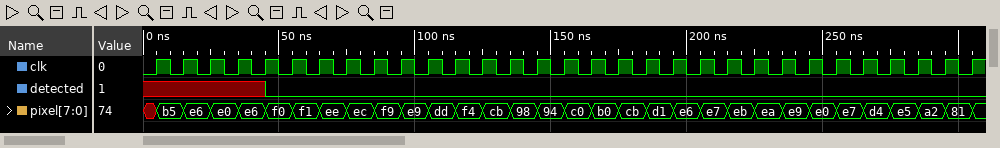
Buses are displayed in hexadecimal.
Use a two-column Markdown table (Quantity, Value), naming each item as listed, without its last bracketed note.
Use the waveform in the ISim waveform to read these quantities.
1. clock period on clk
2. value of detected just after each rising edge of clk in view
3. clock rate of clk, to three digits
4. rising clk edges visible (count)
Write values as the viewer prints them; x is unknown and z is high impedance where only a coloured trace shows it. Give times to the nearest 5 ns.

| Quantity | Value |
|---|---|
| clock period on clk | 10 ns |
| value of detected just after each rising edge of clk in view | x x x x 0 0 0 0 0 0 0 0 0 0 0 0 0 0 0 0 0 0 0 0 0 0 0 0 0 0 0 |
| clock rate of clk, to three digits | 100 MHz |
| rising clk edges visible | 31 |
